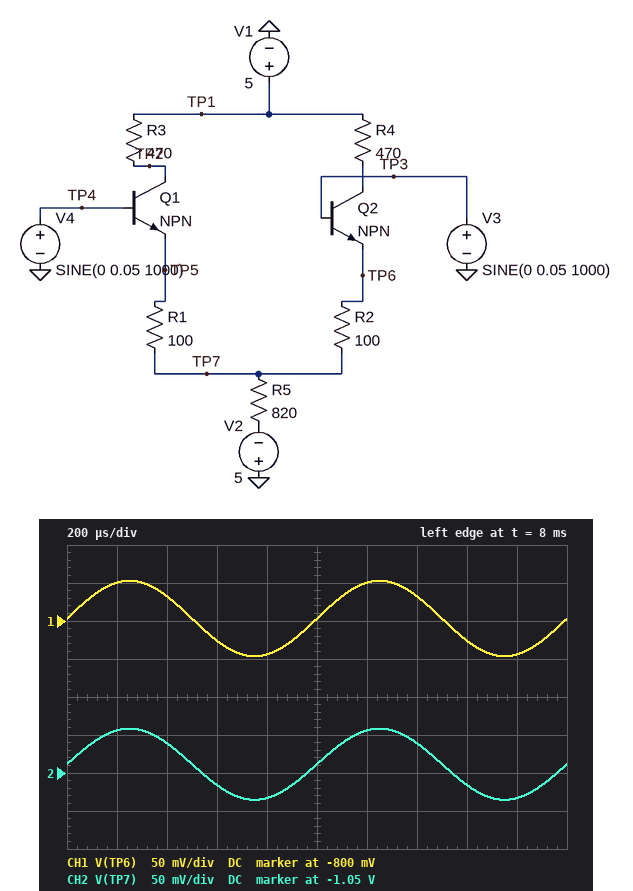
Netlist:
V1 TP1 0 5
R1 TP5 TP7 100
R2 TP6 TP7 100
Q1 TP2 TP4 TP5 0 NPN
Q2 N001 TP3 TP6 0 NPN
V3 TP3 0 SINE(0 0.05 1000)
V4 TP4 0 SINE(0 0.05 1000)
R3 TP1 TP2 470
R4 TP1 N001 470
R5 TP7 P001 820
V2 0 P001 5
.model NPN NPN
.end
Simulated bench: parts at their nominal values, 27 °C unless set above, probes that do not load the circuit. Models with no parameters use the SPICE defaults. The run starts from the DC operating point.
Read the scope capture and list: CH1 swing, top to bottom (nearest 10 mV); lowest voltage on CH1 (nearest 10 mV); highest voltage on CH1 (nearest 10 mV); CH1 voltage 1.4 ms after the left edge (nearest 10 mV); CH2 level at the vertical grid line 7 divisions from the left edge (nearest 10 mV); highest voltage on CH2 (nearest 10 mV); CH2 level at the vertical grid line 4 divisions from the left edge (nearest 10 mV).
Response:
100 mV
-850 mV
-750 mV
-770 mV
-1.01 V
-990 mV
-1.08 V
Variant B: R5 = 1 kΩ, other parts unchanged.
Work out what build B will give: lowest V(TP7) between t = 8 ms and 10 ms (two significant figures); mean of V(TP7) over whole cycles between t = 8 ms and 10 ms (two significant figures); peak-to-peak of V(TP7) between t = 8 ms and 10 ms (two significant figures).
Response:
-1.0 V
-990 mV
95 mV
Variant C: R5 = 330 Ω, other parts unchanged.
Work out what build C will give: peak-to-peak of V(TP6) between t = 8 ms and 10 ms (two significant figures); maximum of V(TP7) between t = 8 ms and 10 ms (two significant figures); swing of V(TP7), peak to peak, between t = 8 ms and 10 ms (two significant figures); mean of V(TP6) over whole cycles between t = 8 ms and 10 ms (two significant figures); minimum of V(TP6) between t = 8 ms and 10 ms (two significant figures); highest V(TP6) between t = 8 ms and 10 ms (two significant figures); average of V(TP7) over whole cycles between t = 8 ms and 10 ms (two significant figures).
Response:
99 mV
-1.3 V
86 mV
-820 mV
-870 mV
-770 mV
-1.4 V
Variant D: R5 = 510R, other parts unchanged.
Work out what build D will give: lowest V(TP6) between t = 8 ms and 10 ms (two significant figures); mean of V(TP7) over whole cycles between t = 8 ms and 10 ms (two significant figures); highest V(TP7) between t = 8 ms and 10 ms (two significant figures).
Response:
-860 mV
-1.2 V
-1.1 V
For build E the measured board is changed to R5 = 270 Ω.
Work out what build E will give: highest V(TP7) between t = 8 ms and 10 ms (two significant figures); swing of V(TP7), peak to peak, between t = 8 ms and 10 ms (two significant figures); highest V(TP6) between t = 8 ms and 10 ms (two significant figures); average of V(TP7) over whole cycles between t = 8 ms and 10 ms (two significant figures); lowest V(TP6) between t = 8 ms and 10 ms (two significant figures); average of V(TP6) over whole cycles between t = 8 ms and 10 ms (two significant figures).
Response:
-1.4 V
84 mV
-770 mV
-1.5 V
-870 mV
-820 mV
